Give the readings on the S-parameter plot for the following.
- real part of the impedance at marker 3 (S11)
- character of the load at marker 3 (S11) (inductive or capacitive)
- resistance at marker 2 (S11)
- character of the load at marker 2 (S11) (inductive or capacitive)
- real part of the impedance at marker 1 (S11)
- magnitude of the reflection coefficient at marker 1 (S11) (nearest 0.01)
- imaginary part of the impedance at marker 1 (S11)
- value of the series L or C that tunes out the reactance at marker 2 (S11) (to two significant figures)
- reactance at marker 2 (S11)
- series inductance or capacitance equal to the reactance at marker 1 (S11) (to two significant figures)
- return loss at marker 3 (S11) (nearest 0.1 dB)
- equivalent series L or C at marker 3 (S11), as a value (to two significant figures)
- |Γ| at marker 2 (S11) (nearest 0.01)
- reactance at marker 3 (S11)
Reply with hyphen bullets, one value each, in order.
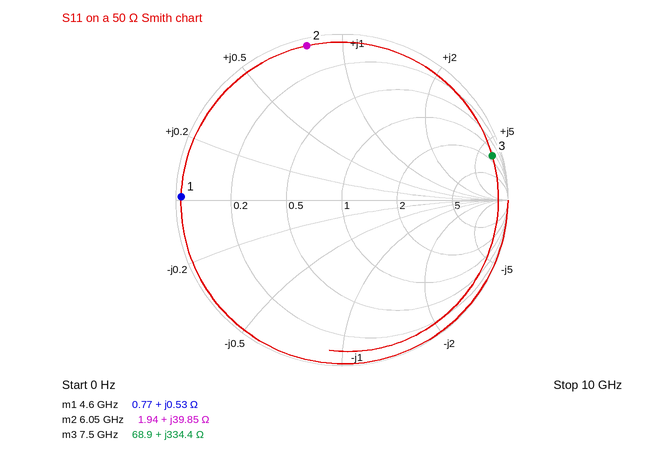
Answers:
- 68.9 Ω
- inductive
- 1.94 Ω
- inductive
- 0.77 Ω
- 0.97
- +0.53 Ω
- 660 fF
- +39.85 Ω
- 18 pH
- 0.5 dB
- 7.1 nH
- 0.95
- +334.4 Ω
